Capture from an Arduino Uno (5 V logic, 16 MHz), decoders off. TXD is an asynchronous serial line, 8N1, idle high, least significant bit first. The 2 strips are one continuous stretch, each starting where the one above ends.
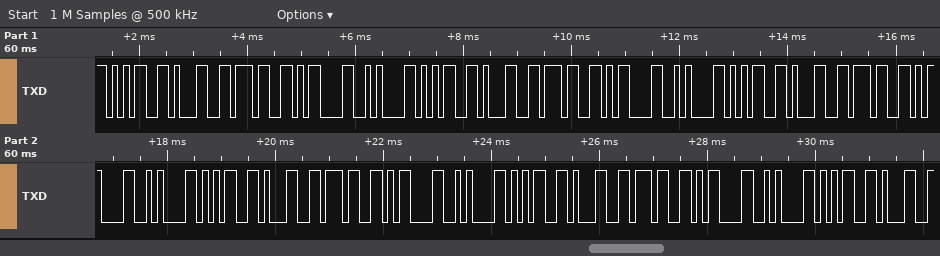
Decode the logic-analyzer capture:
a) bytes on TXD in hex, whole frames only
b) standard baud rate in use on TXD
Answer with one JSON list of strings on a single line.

["35 31 37 0D 0A 35 31 37 0D 0A 35 31 37 0D 0A 35 31 37 0D 0A 35 31 37 0D 0A 35 31", "9600 baud"]
